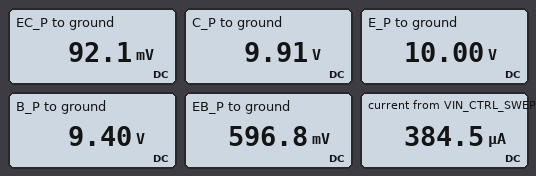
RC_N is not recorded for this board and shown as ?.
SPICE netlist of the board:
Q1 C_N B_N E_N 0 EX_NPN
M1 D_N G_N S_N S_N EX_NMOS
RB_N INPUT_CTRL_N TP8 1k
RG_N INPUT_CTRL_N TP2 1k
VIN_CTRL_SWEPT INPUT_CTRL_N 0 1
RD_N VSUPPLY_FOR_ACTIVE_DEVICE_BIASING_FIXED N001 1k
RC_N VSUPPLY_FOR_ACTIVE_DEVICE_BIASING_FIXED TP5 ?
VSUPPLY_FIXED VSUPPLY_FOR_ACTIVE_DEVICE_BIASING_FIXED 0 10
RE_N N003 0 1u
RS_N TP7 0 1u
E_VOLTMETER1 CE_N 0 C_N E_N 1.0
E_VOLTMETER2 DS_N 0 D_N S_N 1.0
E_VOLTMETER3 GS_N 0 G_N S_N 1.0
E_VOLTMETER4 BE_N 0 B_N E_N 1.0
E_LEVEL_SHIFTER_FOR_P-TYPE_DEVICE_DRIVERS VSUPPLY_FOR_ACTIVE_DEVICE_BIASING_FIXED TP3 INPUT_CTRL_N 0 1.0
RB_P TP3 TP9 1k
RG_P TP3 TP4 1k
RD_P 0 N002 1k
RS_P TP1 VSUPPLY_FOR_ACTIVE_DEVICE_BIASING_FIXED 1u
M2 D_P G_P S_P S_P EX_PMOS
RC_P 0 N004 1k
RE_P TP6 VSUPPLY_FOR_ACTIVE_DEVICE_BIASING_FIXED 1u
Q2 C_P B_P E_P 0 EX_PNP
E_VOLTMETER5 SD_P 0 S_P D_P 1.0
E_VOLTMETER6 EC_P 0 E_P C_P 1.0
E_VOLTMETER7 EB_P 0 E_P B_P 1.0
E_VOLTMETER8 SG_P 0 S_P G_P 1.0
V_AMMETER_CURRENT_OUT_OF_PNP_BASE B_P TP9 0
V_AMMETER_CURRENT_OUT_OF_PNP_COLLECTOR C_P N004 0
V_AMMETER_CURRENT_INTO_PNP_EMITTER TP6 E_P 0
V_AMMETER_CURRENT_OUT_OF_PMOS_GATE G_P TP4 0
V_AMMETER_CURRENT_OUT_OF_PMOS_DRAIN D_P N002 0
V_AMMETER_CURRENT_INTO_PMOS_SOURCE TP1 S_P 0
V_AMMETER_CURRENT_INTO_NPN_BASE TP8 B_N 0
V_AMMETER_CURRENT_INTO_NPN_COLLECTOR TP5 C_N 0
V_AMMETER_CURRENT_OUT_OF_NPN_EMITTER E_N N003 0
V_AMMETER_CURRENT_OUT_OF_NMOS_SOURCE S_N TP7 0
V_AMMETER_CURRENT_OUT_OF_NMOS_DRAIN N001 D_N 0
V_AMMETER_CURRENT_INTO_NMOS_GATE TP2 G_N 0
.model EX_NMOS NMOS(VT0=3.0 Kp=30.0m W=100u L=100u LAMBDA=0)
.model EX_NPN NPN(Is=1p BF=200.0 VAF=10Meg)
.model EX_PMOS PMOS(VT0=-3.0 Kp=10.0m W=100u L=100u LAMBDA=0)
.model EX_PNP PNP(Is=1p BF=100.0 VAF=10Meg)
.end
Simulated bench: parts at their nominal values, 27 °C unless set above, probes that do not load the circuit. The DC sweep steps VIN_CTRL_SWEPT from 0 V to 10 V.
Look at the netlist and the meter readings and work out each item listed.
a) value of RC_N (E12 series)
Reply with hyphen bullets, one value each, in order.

- 470 Ω
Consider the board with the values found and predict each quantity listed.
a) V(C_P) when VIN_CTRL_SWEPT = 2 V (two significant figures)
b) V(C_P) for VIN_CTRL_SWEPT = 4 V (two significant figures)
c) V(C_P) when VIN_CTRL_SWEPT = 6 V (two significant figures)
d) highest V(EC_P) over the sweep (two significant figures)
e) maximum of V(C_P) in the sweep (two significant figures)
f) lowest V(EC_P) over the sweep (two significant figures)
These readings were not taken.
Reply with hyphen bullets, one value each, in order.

- 9.9 V
- 10 V
- 10 V
- 10 V
- 10 V
- 29 mV
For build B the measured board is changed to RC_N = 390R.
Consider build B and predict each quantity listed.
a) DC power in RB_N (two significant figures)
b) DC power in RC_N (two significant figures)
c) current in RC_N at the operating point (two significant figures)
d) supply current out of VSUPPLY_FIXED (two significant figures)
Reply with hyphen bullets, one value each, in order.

- 140 µW
- 250 mW
- 25 mA
- 35 mA
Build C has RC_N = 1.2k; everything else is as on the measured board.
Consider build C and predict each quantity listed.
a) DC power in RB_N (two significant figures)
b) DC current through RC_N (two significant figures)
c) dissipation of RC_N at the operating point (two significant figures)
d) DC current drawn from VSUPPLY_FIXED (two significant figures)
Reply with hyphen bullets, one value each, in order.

- 170 µW
- 8.3 mA
- 82 mW
- 18 mA
